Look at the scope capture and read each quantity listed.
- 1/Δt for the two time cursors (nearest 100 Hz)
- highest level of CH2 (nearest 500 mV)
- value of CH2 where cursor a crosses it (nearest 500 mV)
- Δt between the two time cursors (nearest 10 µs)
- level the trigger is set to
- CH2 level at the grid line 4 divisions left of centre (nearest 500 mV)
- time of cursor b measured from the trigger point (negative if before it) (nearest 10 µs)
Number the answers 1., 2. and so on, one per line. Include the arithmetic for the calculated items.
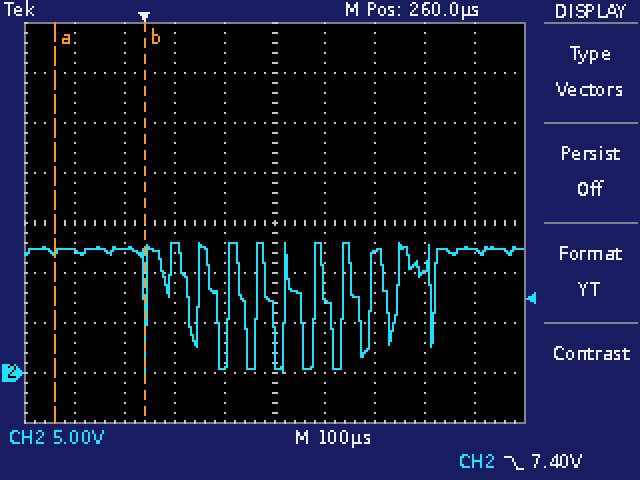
1. 1 / 180 µs ≈ 5.6 kHz
2. 13.0 V
3. 12.0 V
4. 180 µs
5. 7.40 V
6. 12.0 V
7. 0 µs
